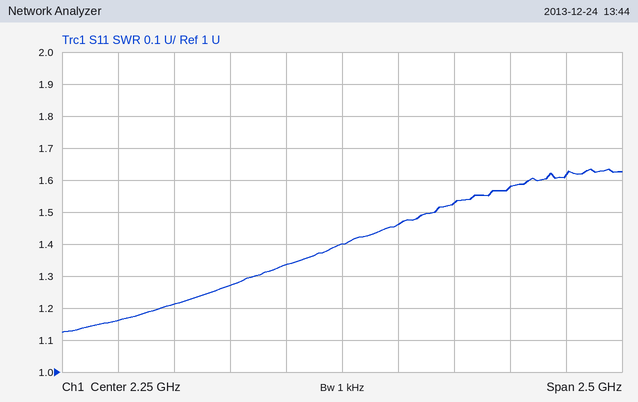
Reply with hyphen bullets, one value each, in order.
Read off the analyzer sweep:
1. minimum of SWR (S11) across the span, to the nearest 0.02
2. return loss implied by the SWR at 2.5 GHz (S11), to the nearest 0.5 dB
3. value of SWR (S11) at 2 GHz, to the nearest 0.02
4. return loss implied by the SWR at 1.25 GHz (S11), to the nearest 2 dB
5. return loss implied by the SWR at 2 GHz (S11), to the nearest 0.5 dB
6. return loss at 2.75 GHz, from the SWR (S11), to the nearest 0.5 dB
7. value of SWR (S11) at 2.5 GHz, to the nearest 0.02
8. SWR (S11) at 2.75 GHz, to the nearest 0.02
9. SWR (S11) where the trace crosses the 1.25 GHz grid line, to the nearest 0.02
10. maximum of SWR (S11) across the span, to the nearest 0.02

- 1.12
- 14.5 dB
- 1.34
- 22 dB
- 17.0 dB
- 13.5 dB
- 1.46
- 1.52
- 1.16
- 1.64
